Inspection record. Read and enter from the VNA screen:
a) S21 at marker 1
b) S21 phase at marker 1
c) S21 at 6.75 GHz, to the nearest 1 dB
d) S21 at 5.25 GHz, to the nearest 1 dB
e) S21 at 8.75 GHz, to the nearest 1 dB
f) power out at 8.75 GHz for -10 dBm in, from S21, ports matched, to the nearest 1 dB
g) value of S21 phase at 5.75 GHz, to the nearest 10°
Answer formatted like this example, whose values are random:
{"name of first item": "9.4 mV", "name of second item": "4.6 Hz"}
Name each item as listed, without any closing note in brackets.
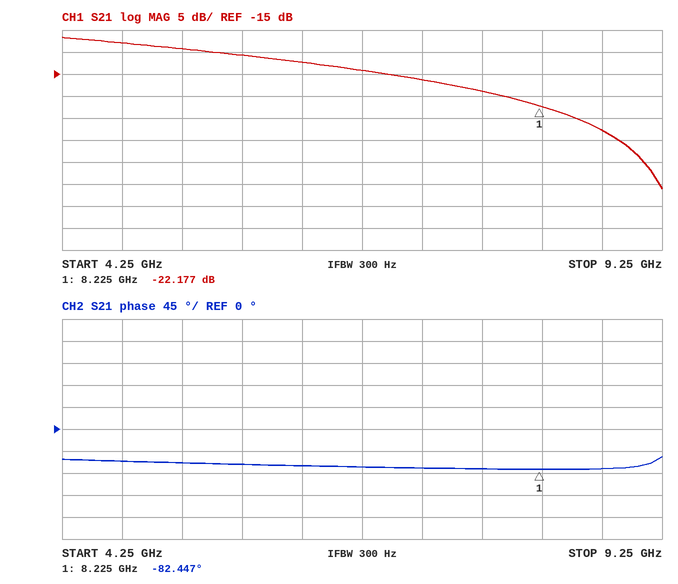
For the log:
{"S21 at marker 1": "-22.177 dB", "S21 phase at marker 1": "-82.447°", "S21 at 6.75 GHz, to the nearest 1 dB": "-14 dB", "S21 at 5.25 GHz, to the nearest 1 dB": "-9 dB", "S21 at 8.75 GHz, to the nearest 1 dB": "-28 dB", "power out at 8.75 GHz for -10 dBm in, from S21, ports matched, to the nearest 1 dB": "-38 dBm", "value of S21 phase at 5.75 GHz, to the nearest 10°": "-70°"}
